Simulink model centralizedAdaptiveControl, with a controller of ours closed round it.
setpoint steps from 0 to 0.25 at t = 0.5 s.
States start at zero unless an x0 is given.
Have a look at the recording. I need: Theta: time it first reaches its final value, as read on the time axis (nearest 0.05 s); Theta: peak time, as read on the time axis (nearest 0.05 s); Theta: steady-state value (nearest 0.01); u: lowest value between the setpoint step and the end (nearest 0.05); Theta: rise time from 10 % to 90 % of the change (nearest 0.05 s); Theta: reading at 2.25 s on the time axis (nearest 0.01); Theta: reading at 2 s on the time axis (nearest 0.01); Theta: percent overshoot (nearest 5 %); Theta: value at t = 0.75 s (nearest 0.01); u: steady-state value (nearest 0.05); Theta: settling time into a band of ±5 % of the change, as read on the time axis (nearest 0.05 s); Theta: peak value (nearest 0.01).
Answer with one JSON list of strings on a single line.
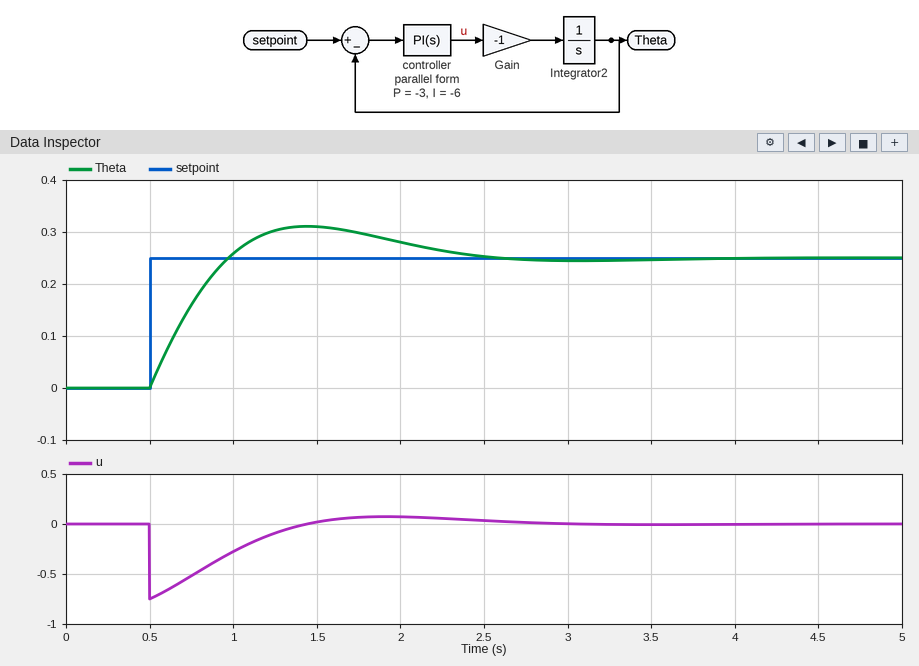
["0.95 s", "1.45 s", "0.25", "-0.75", "0.35 s", "0.26", "0.28", "25 %", "0.16", "0.00", "2.30 s", "0.31"]
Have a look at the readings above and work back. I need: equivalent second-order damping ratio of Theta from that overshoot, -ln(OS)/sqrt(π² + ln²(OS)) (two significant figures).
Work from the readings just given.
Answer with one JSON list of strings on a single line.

["0.40"]
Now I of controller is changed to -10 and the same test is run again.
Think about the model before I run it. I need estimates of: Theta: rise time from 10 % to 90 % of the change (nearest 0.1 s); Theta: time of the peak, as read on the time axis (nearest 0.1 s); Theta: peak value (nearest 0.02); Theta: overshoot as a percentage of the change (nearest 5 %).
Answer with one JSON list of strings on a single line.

["0.3 s", "1.3 s", "0.32", "30 %"]
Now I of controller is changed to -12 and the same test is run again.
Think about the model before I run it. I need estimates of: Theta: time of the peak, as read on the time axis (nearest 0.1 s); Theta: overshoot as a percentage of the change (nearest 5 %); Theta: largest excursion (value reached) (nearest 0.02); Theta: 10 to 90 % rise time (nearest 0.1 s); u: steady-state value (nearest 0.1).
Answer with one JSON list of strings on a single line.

["1.2 s", "35 %", "0.34", "0.3 s", "0.0"]
